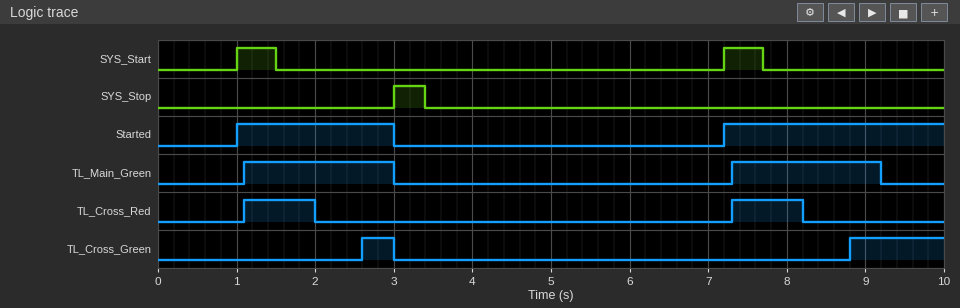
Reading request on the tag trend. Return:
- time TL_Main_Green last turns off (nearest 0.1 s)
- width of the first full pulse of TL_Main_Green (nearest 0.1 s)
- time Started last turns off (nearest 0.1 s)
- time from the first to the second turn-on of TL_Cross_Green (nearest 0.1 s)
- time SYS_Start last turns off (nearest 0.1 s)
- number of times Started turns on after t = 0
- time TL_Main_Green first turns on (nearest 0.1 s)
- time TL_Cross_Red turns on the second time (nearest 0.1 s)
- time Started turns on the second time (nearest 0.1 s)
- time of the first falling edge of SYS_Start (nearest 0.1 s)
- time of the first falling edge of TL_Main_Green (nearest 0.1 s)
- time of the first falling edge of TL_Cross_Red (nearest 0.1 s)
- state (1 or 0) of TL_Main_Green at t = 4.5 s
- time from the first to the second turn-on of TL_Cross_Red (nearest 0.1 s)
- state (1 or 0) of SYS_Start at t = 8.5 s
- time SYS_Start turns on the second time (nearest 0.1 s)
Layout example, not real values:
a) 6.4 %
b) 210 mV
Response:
a) 9.2 s
b) 1.9 s
c) 3.0 s
d) 6.2 s
e) 7.7 s
f) 2
g) 1.1 s
h) 7.3 s
i) 7.2 s
j) 1.5 s
k) 3.0 s
l) 2.0 s
m) 0
n) 6.2 s
o) 0
p) 7.2 s
